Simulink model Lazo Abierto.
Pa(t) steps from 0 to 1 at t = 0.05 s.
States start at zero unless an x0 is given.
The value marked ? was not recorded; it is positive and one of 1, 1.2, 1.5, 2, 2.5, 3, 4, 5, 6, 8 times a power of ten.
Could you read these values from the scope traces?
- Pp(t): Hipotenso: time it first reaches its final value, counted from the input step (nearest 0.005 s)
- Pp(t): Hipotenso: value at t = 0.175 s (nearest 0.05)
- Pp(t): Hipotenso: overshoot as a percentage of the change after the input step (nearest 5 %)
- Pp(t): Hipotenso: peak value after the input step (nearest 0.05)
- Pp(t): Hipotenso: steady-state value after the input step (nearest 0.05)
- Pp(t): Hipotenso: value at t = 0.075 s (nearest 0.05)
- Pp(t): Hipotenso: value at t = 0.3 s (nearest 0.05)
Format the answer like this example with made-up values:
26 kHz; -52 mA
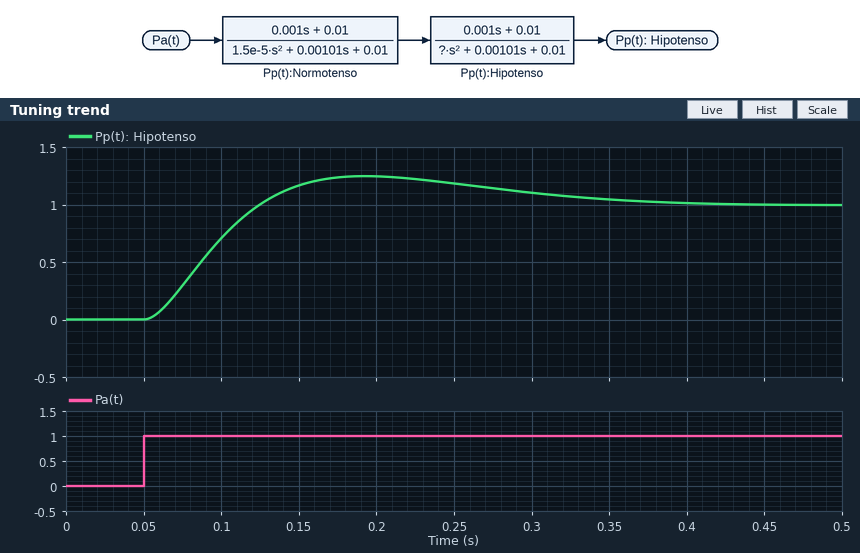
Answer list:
0.075 s; 1.25; 25 %; 1.25; 1.00; 0.30; 1.10
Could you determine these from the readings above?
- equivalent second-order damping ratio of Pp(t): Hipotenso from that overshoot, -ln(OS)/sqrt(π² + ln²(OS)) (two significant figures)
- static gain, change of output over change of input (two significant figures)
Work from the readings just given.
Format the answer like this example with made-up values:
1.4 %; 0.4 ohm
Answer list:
0.40; 1.0
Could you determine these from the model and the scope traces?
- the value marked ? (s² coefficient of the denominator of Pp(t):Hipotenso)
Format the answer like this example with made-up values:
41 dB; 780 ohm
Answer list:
4e-05
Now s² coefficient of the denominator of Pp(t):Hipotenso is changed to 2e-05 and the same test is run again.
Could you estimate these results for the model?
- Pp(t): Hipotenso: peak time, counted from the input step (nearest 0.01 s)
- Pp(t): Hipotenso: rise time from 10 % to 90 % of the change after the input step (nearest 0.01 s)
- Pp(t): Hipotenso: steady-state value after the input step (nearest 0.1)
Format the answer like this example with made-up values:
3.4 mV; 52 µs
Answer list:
0.10 s; 0.04 s; 1.0
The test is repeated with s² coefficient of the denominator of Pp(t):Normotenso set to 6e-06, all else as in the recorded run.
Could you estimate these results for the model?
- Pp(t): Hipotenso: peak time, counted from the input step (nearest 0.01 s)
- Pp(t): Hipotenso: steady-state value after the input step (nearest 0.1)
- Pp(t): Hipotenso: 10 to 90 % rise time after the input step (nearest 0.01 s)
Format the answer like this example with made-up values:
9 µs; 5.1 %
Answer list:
0.14 s; 1.0; 0.05 s
